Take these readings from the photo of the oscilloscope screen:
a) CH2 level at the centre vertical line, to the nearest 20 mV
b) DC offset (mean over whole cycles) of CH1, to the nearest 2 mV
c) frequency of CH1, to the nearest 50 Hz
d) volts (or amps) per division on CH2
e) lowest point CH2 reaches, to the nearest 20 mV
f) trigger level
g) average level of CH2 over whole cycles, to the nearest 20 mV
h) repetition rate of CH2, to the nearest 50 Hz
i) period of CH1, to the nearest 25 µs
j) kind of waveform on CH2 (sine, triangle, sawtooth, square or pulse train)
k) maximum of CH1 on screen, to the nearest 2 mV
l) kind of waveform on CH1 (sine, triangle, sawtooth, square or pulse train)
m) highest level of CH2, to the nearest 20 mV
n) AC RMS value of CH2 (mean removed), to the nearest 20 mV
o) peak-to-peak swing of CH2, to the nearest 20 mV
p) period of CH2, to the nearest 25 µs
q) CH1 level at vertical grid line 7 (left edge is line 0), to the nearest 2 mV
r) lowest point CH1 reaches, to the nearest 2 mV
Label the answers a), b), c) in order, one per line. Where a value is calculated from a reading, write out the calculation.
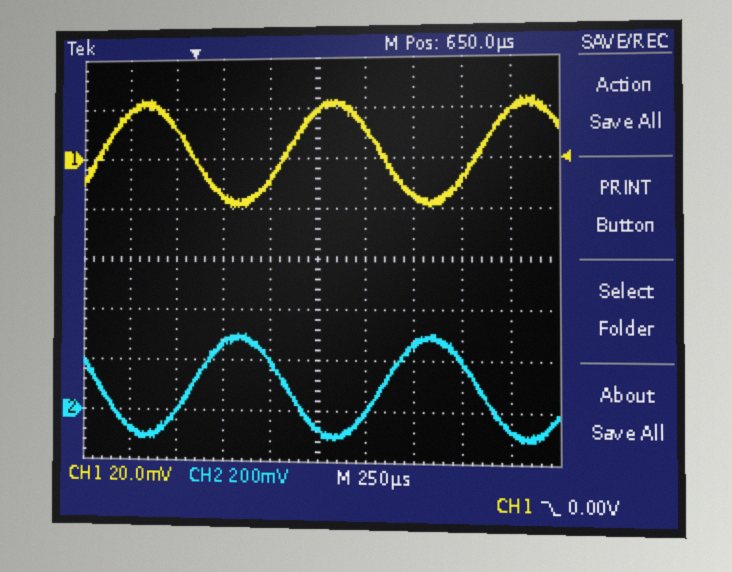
a) -60 mV
b) (24 mV + (-20 mV)) / 2 ≈ 2 mV
c) 1 / 1.000 ms ≈ 1.00 kHz
d) 200 mV
e) -120 mV
f) 0.00 V
g) (300 mV + (-120 mV)) / 2 ≈ 90.0 mV, so 100 mV to the nearest 20 mV
h) 1 / 1.000 ms ≈ 1.00 kHz
i) 1.000 ms
j) sine
k) 24 mV
l) sine
m) 300 mV
n) 420 mV / (2√2) ≈ 148 mV, so 140 mV to the nearest 20 mV
o) 300 mV − (-120 mV) = 420 mV
p) 1.000 ms
q) -14 mV
r) -20 mV
